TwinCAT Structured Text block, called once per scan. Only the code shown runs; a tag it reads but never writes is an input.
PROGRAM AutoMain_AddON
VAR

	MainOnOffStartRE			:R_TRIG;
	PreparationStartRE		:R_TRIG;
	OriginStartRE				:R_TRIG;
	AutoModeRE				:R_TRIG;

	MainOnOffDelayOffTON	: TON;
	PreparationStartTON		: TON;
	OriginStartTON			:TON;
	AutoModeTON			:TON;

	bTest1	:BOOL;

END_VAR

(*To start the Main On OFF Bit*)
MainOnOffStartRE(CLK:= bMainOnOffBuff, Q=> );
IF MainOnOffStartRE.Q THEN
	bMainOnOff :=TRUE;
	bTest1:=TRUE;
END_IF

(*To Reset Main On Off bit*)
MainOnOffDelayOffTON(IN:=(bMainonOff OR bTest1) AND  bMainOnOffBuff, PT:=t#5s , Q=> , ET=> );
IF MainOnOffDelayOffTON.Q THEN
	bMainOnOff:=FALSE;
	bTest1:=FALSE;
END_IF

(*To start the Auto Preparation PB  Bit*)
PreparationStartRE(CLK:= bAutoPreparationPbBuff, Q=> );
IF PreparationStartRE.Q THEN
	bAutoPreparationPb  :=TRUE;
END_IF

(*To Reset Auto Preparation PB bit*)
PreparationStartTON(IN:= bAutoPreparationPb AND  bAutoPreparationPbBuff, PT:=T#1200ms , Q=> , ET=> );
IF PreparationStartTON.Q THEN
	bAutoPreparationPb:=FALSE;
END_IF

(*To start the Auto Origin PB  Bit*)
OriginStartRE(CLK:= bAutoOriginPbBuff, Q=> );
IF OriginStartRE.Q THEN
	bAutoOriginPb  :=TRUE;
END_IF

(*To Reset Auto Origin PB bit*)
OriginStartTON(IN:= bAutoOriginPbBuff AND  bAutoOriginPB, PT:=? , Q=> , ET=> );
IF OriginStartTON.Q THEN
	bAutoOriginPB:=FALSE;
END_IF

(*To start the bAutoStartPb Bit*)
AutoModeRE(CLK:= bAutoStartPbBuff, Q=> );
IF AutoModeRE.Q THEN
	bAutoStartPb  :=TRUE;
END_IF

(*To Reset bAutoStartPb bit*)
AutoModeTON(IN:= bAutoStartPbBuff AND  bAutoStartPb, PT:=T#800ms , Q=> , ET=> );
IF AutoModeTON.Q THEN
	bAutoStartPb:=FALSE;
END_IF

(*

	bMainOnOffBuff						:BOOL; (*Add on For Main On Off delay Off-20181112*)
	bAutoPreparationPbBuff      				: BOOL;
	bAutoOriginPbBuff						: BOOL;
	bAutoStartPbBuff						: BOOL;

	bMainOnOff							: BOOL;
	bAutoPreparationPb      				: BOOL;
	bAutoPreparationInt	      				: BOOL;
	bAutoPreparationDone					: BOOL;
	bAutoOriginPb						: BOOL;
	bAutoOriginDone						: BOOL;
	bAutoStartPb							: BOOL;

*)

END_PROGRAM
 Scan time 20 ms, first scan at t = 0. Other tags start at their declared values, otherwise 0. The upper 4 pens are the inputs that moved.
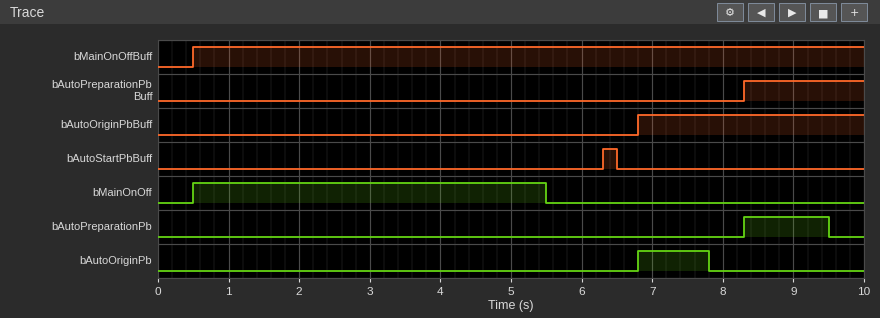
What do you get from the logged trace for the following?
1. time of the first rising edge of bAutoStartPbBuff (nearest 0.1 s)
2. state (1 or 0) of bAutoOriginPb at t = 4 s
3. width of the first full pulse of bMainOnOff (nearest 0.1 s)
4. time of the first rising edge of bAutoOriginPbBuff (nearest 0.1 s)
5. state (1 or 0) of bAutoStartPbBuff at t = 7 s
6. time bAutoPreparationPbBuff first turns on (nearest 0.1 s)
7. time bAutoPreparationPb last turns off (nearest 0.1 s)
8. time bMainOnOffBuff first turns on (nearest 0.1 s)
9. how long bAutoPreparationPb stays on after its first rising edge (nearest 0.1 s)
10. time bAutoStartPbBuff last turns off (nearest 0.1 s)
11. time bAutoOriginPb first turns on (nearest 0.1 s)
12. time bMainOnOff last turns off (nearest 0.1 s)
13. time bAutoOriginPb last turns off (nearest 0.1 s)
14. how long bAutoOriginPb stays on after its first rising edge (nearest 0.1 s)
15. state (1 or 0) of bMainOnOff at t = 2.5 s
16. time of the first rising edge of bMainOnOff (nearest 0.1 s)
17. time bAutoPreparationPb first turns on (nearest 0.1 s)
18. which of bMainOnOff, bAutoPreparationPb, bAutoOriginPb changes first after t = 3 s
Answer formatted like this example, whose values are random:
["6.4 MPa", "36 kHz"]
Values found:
["6.3 s", "0", "5.0 s", "6.8 s", "0", "8.3 s", "9.5 s", "0.5 s", "1.2 s", "6.5 s", "6.8 s", "5.5 s", "7.8 s", "1.0 s", "1", "0.5 s", "8.3 s", "bMainOnOff"]
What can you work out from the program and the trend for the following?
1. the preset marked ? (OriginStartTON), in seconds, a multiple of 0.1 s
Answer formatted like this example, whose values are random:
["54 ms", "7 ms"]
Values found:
["1.0 s"]
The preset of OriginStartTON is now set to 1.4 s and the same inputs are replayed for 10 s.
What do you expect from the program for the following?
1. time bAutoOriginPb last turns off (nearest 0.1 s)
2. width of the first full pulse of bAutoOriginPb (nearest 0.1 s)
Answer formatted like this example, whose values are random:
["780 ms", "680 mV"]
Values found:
["8.2 s", "1.4 s"]
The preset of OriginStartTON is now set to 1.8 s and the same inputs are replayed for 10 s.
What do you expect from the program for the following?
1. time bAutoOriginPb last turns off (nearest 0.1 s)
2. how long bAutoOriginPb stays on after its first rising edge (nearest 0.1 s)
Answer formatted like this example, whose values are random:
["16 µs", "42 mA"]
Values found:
["8.6 s", "1.8 s"]
